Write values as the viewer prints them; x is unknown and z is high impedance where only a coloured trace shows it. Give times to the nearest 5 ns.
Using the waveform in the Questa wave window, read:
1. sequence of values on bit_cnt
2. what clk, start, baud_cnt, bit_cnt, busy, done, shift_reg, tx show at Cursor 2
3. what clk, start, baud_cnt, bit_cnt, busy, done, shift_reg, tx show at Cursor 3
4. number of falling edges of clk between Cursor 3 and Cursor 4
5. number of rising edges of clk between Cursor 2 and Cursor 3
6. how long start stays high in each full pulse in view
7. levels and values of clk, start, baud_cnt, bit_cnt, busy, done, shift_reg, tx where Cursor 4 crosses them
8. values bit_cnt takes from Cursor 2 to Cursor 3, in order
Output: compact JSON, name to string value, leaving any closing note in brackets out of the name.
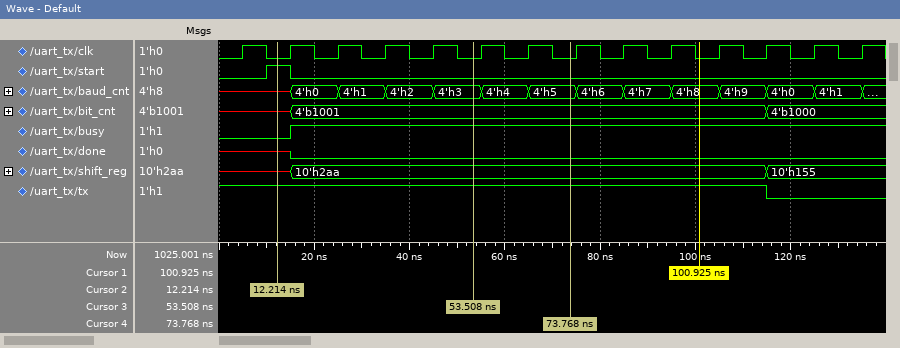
{"sequence of values on bit_cnt": "x, 4'b1001, 4'b1000", "what clk, start, baud_cnt, bit_cnt, busy, done, shift_reg, tx show at Cursor 2": "clk=0, start=1, baud_cnt=x, bit_cnt=x, busy=0, done=x, shift_reg=x, tx=1", "what clk, start, baud_cnt, bit_cnt, busy, done, shift_reg, tx show at Cursor 3": "clk=0, start=0, baud_cnt=4'h3, bit_cnt=4'b1001, busy=1, done=0, shift_reg=10'h2aa, tx=1", "number of falling edges of clk between Cursor 3 and Cursor 4": "2", "number of rising edges of clk between Cursor 2 and Cursor 3": "4", "how long start stays high in each full pulse in view": "5 ns", "levels and values of clk, start, baud_cnt, bit_cnt, busy, done, shift_reg, tx where Cursor 4 crosses them": "clk=0, start=0, baud_cnt=4'h5, bit_cnt=4'b1001, busy=1, done=0, shift_reg=10'h2aa, tx=1", "values bit_cnt takes from Cursor 2 to Cursor 3, in order": "x, 4'b1001"}
